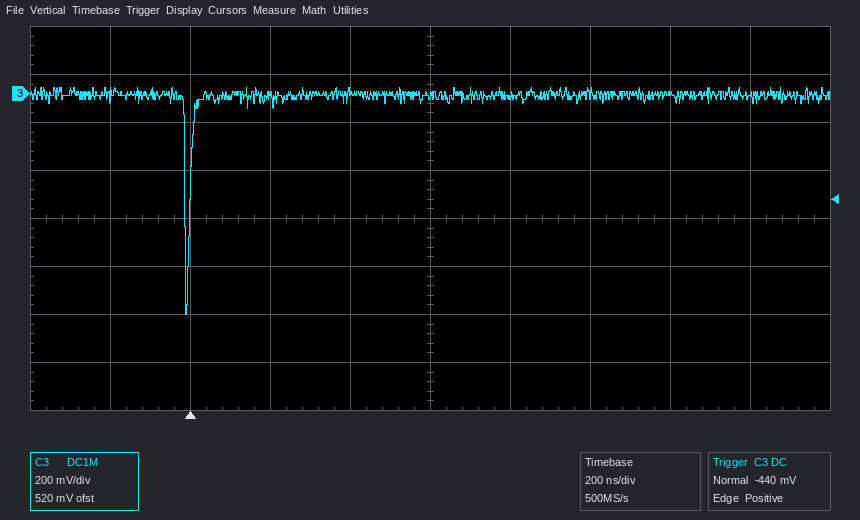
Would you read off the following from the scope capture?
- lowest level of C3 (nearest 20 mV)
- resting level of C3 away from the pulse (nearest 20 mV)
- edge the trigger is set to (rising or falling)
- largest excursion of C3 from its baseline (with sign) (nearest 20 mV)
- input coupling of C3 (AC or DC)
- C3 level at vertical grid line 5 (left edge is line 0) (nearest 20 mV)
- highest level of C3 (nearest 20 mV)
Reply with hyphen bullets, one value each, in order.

- -920 mV
- 0 mV
- rising
- -920 mV
- DC
- 0 mV
- 20 mV
